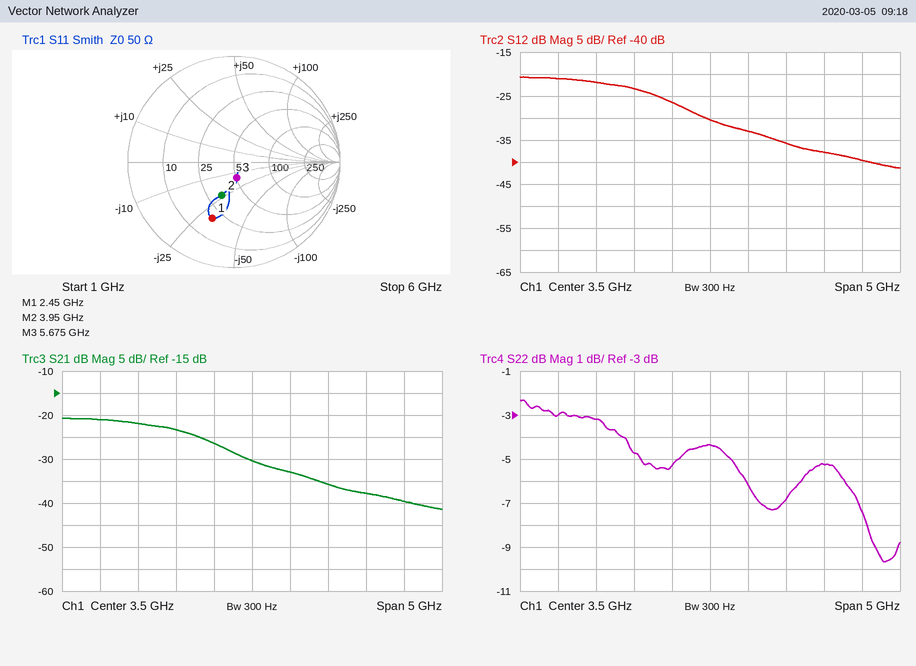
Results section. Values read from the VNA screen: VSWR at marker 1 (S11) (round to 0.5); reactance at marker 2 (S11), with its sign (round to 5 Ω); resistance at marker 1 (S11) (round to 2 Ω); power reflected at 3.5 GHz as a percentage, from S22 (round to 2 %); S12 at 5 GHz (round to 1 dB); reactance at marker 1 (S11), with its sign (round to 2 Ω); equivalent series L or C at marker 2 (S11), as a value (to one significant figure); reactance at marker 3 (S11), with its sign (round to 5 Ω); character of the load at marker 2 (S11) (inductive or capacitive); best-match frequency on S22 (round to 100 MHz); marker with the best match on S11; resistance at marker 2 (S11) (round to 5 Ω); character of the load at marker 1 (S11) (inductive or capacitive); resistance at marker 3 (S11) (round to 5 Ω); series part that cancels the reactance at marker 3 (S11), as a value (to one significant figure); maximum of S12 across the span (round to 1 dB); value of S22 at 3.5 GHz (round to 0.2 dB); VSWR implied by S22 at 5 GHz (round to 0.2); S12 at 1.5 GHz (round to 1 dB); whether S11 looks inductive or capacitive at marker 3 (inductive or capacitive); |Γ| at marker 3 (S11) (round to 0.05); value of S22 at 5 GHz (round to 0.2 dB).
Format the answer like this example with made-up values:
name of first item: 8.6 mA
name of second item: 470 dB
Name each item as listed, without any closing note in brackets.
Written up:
VSWR at marker 1 (S11): 3.5
reactance at marker 2 (S11), with its sign: -25 Ω
resistance at marker 1 (S11): 20 Ω
power reflected at 3.5 GHz as a percentage, from S22: 36 %
S12 at 5 GHz: -38 dB
reactance at marker 1 (S11), with its sign: -30 Ω
equivalent series L or C at marker 2 (S11), as a value: 2 pF
reactance at marker 3 (S11), with its sign: -15 Ω
character of the load at marker 2 (S11): capacitive
best-match frequency on S22: 5.8 GHz
marker with the best match on S11: marker 3
resistance at marker 2 (S11): 35 Ω
character of the load at marker 1 (S11): capacitive
resistance at marker 3 (S11): 50 Ω
series part that cancels the reactance at marker 3 (S11), as a value: 400 pH
maximum of S12 across the span: -21 dB
value of S22 at 3.5 GHz: -4.4 dB
VSWR implied by S22 at 5 GHz: 3.4
S12 at 1.5 GHz: -21 dB
whether S11 looks inductive or capacitive at marker 3: capacitive
|Γ| at marker 3 (S11): 0.15
value of S22 at 5 GHz: -5.2 dB
